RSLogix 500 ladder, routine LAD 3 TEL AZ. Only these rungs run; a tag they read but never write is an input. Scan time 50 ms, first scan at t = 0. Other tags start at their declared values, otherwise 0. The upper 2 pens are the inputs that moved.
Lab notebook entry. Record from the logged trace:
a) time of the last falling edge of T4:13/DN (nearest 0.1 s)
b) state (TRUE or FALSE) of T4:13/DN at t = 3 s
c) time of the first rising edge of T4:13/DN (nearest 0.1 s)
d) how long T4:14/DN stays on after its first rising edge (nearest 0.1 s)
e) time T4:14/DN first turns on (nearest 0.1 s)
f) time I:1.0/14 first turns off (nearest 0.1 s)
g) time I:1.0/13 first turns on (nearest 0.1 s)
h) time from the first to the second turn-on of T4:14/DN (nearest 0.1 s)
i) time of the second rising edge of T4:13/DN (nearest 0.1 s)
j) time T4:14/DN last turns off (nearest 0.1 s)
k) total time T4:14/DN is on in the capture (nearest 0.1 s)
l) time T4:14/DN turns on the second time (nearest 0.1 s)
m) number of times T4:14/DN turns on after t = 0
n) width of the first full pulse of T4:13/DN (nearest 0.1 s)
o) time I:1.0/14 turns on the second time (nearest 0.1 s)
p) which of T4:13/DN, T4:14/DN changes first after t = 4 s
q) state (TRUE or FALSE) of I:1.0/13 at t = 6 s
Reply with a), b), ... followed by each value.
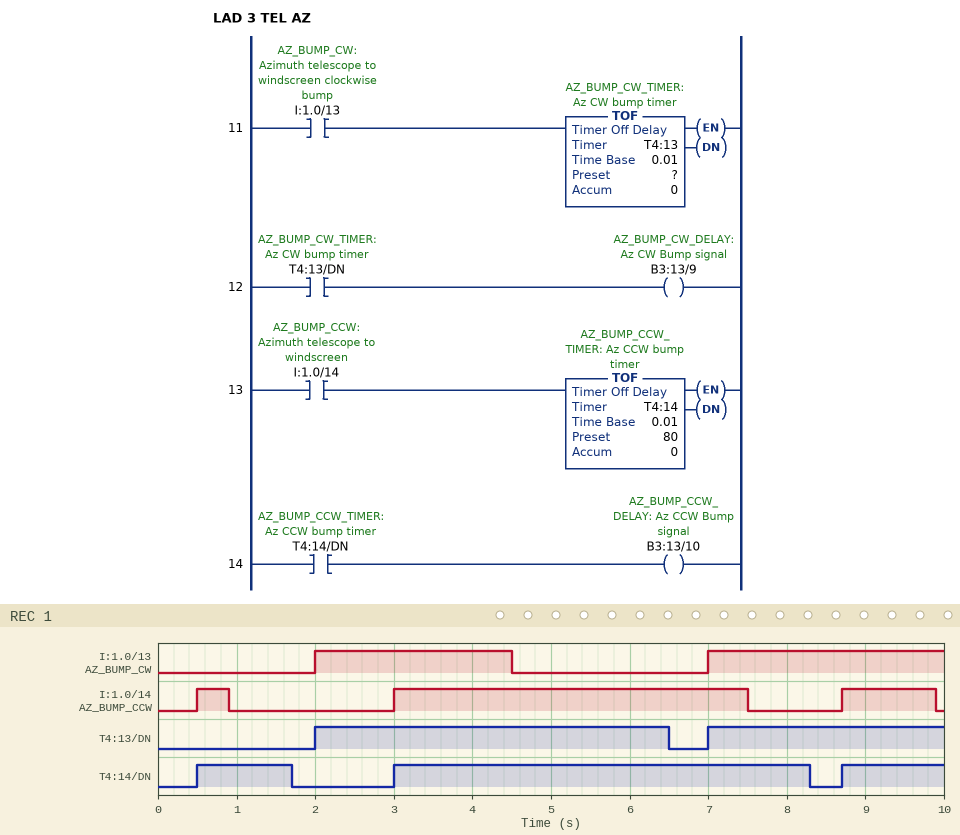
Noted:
a) 6.5 s
b) TRUE
c) 2.0 s
d) 1.2 s
e) 0.5 s
f) 0.9 s
g) 2.0 s
h) 2.5 s
i) 7.0 s
j) 8.3 s
k) 7.8 s
l) 3.0 s
m) 3
n) 4.5 s
o) 3.0 s
p) T4:13/DN
q) FALSE
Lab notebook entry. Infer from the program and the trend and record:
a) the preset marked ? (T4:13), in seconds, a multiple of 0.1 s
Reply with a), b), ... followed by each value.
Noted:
a) 2.0 s
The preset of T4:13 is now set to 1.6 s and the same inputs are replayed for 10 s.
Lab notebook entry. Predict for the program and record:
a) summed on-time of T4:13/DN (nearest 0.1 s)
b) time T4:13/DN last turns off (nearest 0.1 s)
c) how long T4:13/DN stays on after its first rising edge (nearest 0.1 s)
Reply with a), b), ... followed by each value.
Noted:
a) 7.1 s
b) 6.1 s
c) 4.1 s
